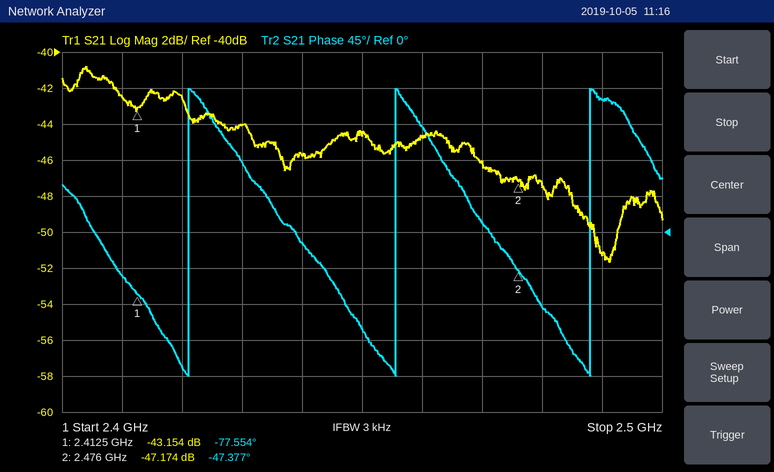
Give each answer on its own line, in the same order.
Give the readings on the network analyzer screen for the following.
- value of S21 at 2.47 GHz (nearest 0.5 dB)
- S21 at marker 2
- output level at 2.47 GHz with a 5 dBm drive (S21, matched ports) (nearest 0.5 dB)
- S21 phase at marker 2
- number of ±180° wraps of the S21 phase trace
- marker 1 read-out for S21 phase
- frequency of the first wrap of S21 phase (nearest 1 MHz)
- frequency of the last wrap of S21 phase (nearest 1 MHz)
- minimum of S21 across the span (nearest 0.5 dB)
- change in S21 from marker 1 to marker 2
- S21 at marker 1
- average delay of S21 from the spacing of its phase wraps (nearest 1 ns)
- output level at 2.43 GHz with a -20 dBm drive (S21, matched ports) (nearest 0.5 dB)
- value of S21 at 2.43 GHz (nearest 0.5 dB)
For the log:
-46.0 dB
-47.174 dB
-41.0 dBm
-47.377°
3
-77.554°
2.421 GHz
2.488 GHz
-51.5 dB
-4.020 dB
-43.154 dB
30 ns
-64.0 dBm
-44.0 dB
